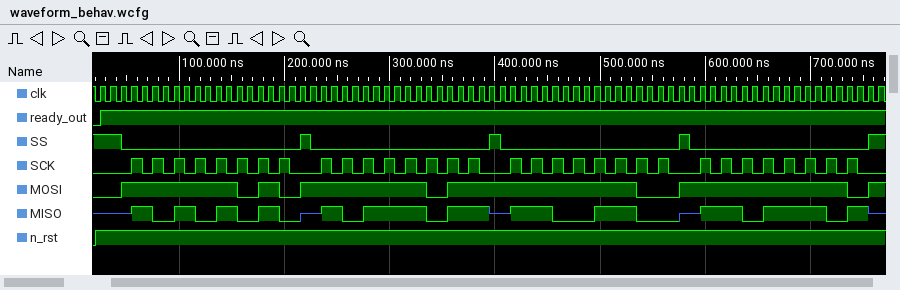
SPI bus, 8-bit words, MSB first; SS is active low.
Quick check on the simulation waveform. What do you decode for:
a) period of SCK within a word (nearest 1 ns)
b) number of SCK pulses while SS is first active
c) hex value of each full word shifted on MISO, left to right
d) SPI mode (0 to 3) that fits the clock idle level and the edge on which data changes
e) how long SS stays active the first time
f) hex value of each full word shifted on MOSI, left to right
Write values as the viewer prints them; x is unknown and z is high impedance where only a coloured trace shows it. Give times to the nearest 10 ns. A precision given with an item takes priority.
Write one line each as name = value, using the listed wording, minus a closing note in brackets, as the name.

period of SCK within a word = 20 ns
number of SCK pulses while SS is first active = 8
hex value of each full word shifted on MISO, left to right = AA, BB, CC, DD
SPI mode (0 to 3) that fits the clock idle level and the edge on which data changes = 1
how long SS stays active the first time = 170 ns
hex value of each full word shifted on MOSI, left to right = FA, FB, FC, FE
